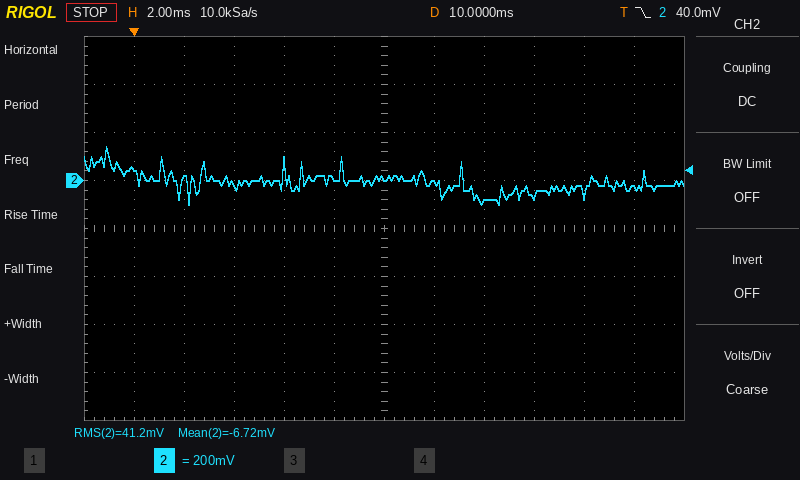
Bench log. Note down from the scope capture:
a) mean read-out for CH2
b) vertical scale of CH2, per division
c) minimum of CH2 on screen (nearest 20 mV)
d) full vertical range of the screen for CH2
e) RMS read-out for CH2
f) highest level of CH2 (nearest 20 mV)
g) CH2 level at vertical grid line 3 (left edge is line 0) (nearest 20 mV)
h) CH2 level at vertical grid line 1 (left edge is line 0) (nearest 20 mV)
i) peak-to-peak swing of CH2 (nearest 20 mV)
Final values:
-6.72 mV
200 mV
-100 mV
1.6 V
41.2 mV
140 mV
-20 mV
40 mV
240 mV
